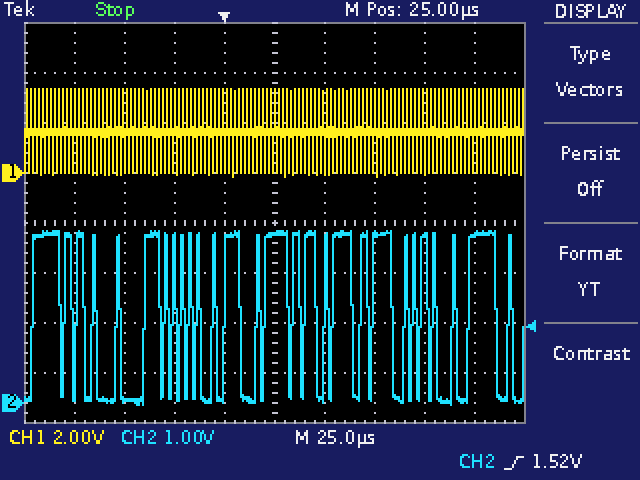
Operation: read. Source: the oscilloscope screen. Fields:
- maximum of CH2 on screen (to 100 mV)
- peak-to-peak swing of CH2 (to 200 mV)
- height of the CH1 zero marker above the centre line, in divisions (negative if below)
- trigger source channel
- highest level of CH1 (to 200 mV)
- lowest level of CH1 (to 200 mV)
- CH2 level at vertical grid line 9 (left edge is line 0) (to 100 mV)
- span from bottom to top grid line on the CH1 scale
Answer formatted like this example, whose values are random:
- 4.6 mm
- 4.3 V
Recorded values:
- 3.4 V
- 3.4 V
- +1.0 div
- CH2
- 3.4 V
- -200 mV
- 3.4 V
- 16 V
